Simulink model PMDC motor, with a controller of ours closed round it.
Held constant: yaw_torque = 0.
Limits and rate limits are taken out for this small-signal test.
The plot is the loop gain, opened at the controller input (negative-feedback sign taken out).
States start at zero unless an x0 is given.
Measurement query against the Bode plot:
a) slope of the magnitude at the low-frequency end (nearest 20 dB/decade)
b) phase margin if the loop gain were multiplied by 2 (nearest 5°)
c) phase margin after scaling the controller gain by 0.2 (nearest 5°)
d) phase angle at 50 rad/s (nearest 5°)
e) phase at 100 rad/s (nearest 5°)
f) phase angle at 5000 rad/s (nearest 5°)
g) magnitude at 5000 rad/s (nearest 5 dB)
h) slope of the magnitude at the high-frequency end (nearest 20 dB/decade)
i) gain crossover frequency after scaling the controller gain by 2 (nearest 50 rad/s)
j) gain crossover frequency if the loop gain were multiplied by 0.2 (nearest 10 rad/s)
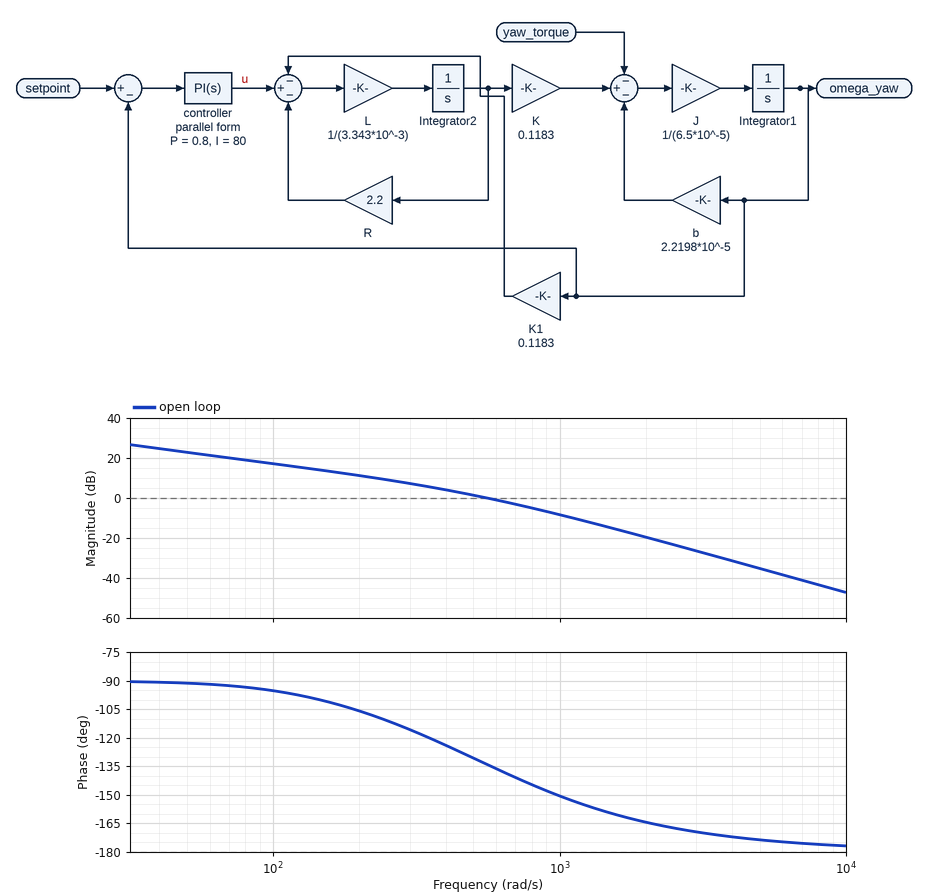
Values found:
-20 dB/decade
35°
80°
-90°
-95°
-175°
-35 dB
-40 dB/decade
850 rad/s
150 rad/s
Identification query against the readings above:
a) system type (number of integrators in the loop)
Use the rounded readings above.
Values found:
1
